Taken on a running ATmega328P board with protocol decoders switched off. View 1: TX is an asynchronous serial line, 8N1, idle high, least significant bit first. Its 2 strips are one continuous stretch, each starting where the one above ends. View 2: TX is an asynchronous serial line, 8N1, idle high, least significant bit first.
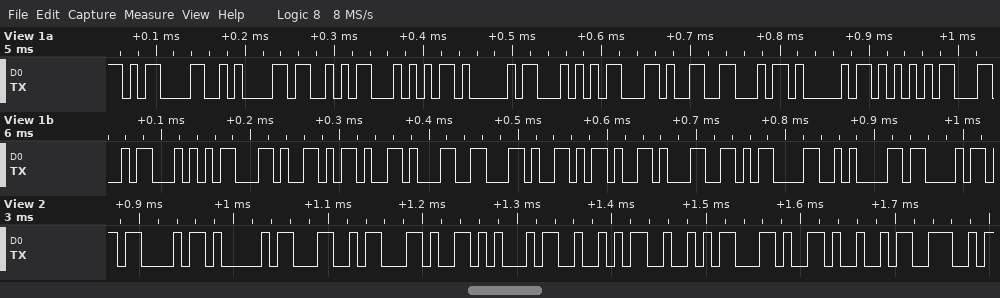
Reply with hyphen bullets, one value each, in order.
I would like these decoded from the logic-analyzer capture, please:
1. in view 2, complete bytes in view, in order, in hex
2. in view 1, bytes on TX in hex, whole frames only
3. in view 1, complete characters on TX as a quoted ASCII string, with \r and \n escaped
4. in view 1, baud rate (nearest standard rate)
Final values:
- 0x43 0x41 0x4C 0x2C 0x45 0x52 0x52 0x2C 0x49 0x4E
- 0D 0A 53 54 41 54 2C 46 41 55 4C 54 2C 2D 31 2C 2D 31 0D 0A 43
- "\r\nSTAT,FAULT,-1,-1\r\nC"
- 115200 baud
